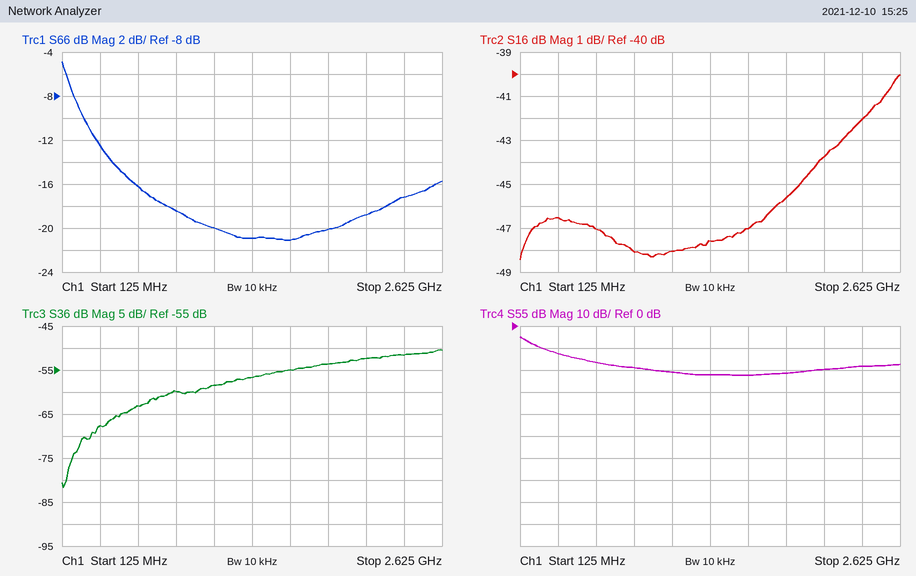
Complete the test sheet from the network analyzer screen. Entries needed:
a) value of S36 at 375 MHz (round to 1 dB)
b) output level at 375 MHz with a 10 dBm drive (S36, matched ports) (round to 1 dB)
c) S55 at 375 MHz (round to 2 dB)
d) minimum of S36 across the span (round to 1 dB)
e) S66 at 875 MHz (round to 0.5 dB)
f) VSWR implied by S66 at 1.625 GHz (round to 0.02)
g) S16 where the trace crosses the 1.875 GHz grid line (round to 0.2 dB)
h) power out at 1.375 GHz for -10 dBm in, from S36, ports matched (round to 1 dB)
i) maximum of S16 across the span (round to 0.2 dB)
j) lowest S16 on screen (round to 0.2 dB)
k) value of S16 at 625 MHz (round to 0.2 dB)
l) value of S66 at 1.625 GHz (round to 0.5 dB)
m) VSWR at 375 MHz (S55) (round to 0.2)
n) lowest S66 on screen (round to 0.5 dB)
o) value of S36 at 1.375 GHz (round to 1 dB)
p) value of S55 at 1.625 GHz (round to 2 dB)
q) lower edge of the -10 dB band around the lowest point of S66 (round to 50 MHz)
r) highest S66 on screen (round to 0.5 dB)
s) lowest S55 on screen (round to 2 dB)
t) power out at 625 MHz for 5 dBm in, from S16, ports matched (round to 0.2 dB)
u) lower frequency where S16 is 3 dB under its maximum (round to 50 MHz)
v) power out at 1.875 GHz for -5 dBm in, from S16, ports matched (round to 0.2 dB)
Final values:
-68 dB
-58 dBm
-12 dB
-82 dB
-18.5 dB
1.20
-45.6 dB
-67 dBm
-40.0 dB
-48.4 dB
-47.0 dB
-21.0 dB
1.6
-21.0 dB
-57 dB
-22 dB
250 MHz
-5.0 dB
-22 dB
-42.0 dBm
2.25 GHz
-50.6 dBm
